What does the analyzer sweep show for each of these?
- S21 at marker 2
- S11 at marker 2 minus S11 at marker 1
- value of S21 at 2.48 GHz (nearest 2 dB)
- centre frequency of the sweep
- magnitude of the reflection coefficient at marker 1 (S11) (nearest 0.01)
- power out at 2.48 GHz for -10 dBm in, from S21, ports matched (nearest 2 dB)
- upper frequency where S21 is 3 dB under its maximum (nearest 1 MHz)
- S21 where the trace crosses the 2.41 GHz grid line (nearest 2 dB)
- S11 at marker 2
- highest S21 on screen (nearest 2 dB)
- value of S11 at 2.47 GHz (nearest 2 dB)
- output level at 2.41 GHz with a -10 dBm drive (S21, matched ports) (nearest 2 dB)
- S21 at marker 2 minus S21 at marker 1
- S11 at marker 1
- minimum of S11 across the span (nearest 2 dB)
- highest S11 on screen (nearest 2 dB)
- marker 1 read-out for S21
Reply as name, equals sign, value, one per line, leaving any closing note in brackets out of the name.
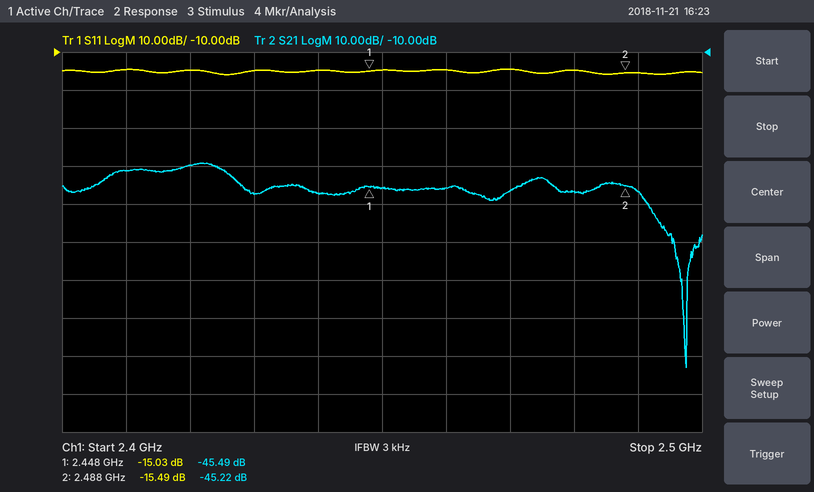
S21 at marker 2 = -45.22 dB
S11 at marker 2 minus S11 at marker 1 = -0.46 dB
value of S21 at 2.48 GHz = -46 dB
centre frequency of the sweep = 2.45 GHz
magnitude of the reflection coefficient at marker 1 (S11) = 0.18
power out at 2.48 GHz for -10 dBm in, from S21, ports matched = -56 dBm
upper frequency where S21 is 3 dB under its maximum = 2.426 GHz
S21 where the trace crosses the 2.41 GHz grid line = -42 dB
S11 at marker 2 = -15.49 dB
highest S21 on screen = -40 dB
value of S11 at 2.47 GHz = -14 dB
output level at 2.41 GHz with a -10 dBm drive (S21, matched ports) = -52 dBm
S21 at marker 2 minus S21 at marker 1 = 0.27 dB
S11 at marker 1 = -15.03 dB
minimum of S11 across the span = -16 dB
highest S11 on screen = -14 dB
marker 1 read-out for S21 = -45.49 dB
